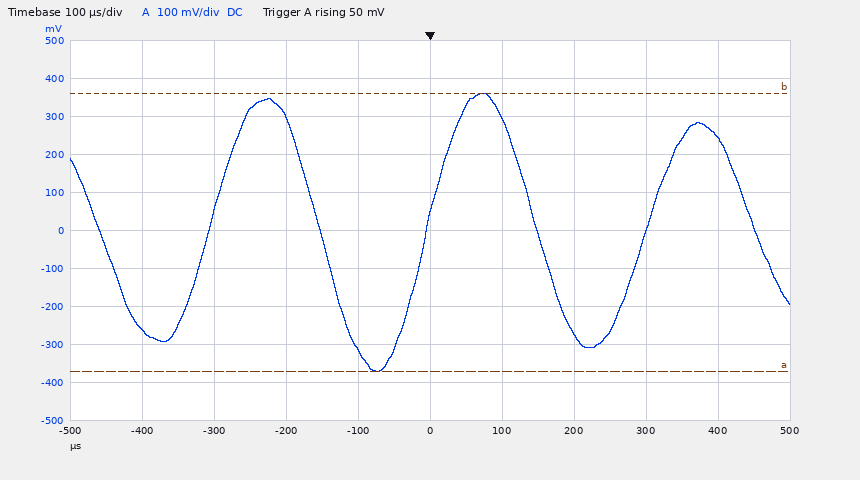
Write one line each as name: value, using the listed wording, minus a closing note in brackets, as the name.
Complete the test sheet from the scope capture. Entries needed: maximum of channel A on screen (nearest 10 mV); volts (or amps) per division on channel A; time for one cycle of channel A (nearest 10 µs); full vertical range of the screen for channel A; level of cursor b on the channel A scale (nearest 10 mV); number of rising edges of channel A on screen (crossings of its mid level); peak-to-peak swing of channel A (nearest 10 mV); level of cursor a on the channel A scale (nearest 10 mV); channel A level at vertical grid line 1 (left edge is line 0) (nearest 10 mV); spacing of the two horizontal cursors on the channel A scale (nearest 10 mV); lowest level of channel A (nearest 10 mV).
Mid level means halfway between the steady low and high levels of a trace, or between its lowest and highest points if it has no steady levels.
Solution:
maximum of channel A on screen: 360 mV
volts (or amps) per division on channel A: 100 mV
time for one cycle of channel A: 300 µs
full vertical range of the screen for channel A: 1 V
level of cursor b on the channel A scale: 360 mV
number of rising edges of channel A on screen: 3
peak-to-peak swing of channel A: 730 mV
level of cursor a on the channel A scale: -370 mV
channel A level at vertical grid line 1 (left edge is line 0): -260 mV
spacing of the two horizontal cursors on the channel A scale: 730 mV
lowest level of channel A: -370 mV
